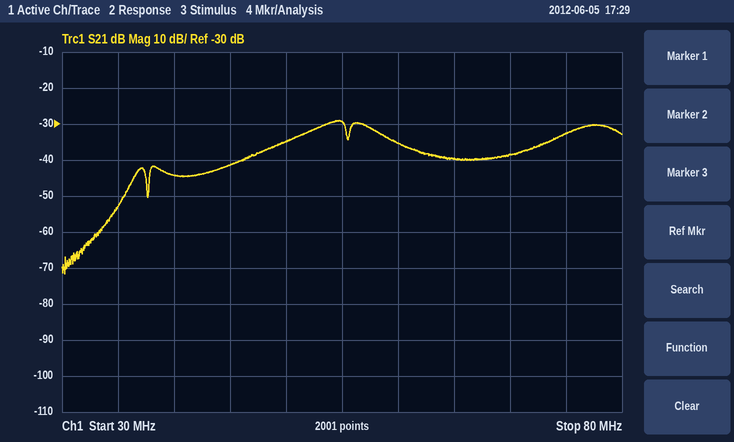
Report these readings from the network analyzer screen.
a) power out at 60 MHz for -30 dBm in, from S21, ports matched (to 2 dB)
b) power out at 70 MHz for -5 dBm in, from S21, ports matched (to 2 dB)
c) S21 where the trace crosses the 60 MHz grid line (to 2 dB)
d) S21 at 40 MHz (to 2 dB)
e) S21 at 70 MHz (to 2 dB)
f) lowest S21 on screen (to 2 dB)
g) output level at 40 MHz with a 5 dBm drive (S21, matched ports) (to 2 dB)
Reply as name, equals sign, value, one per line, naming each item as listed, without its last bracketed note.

power out at 60 MHz for -30 dBm in, from S21, ports matched = -66 dBm
power out at 70 MHz for -5 dBm in, from S21, ports matched = -44 dBm
S21 where the trace crosses the 60 MHz grid line = -36 dB
S21 at 40 MHz = -44 dB
S21 at 70 MHz = -38 dB
lowest S21 on screen = -72 dB
output level at 40 MHz with a 5 dBm drive (S21, matched ports) = -40 dBm
